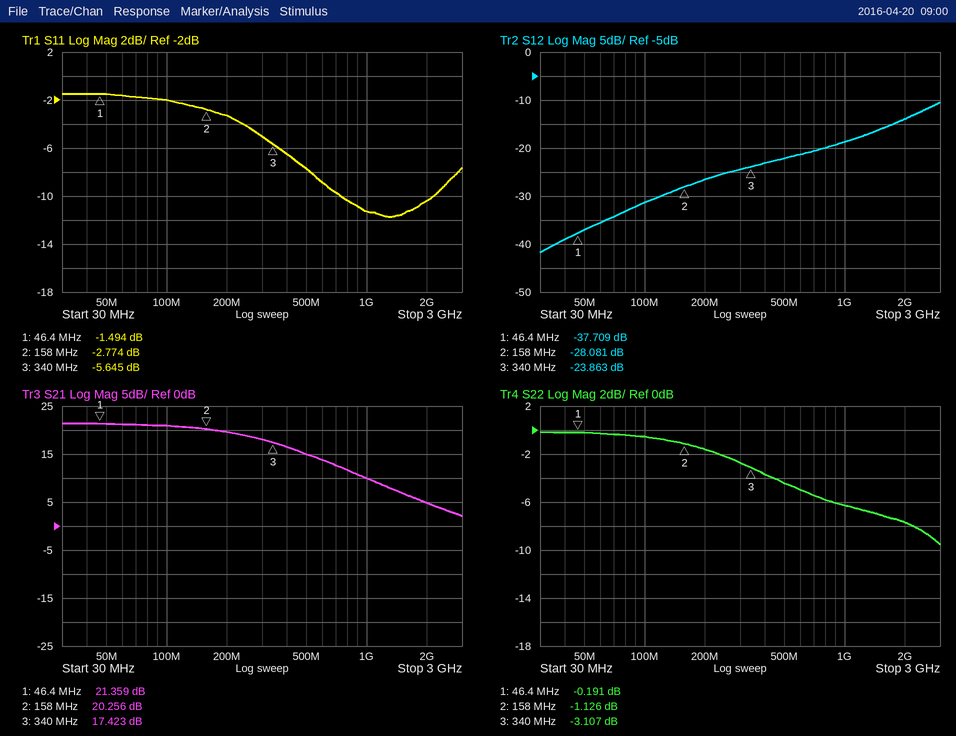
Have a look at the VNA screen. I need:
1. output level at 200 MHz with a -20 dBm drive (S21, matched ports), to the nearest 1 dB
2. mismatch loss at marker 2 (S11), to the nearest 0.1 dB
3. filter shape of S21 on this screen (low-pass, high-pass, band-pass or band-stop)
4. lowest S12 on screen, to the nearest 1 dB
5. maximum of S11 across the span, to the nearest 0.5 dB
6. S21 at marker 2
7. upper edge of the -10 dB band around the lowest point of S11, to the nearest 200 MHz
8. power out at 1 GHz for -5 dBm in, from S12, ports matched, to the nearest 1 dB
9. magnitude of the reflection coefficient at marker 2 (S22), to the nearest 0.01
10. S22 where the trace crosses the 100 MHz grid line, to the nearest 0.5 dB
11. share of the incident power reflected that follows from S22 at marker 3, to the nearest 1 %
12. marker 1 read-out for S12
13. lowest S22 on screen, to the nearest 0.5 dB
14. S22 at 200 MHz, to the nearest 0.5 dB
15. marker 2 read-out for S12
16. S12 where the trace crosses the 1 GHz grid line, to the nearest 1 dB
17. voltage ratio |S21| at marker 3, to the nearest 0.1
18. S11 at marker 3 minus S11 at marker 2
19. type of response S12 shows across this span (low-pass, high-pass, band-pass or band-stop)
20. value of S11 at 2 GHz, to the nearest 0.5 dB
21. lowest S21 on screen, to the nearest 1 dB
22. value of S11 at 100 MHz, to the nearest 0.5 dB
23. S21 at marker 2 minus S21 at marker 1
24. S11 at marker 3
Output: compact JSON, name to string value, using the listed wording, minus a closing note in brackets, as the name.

{"output level at 200 MHz with a -20 dBm drive (S21, matched ports), to the nearest 1 dB": "0 dBm", "mismatch loss at marker 2 (S11), to the nearest 0.1 dB": "3.3 dB", "filter shape of S21 on this screen": "low-pass", "lowest S12 on screen, to the nearest 1 dB": "-42 dB", "maximum of S11 across the span, to the nearest 0.5 dB": "-1.5 dB", "S21 at marker 2": "20.256 dB", "upper edge of the -10 dB band around the lowest point of S11, to the nearest 200 MHz": "2.2 GHz", "power out at 1 GHz for -5 dBm in, from S12, ports matched, to the nearest 1 dB": "-24 dBm", "magnitude of the reflection coefficient at marker 2 (S22), to the nearest 0.01": "0.88", "S22 where the trace crosses the 100 MHz grid line, to the nearest 0.5 dB": "-0.5 dB", "share of the incident power reflected that follows from S22 at marker 3, to the nearest 1 %": "49 %", "marker 1 read-out for S12": "-37.709 dB", "lowest S22 on screen, to the nearest 0.5 dB": "-9.5 dB", "S22 at 200 MHz, to the nearest 0.5 dB": "-1.5 dB", "marker 2 read-out for S12": "-28.081 dB", "S12 where the trace crosses the 1 GHz grid line, to the nearest 1 dB": "-19 dB", "voltage ratio |S21| at marker 3, to the nearest 0.1": "7.4", "S11 at marker 3 minus S11 at marker 2": "-2.871 dB", "type of response S12 shows across this span": "high-pass", "value of S11 at 2 GHz, to the nearest 0.5 dB": "-10.5 dB", "lowest S21 on screen, to the nearest 1 dB": "2 dB", "value of S11 at 100 MHz, to the nearest 0.5 dB": "-2.0 dB", "S21 at marker 2 minus S21 at marker 1": "-1.103 dB", "S11 at marker 3": "-5.645 dB"}
